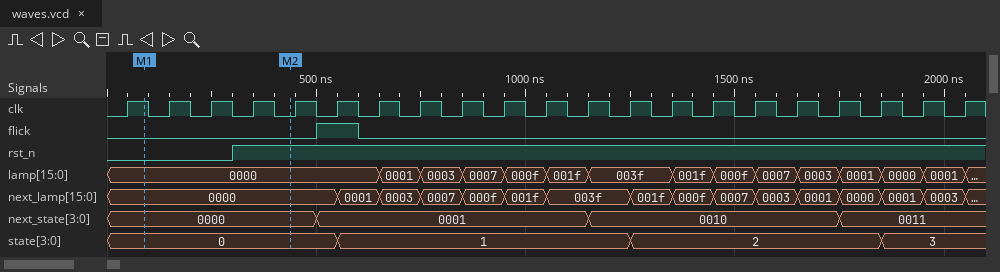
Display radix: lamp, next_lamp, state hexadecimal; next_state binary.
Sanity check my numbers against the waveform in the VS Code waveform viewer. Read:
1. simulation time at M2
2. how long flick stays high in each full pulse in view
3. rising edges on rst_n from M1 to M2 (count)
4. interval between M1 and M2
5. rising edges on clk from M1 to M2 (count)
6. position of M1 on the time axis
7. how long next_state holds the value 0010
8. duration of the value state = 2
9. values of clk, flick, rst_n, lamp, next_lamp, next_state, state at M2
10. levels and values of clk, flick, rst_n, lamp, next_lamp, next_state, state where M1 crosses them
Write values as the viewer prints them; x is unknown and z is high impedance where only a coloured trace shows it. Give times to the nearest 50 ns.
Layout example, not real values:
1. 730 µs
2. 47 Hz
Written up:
1. 450 ns
2. 100 ns
3. 1
4. 350 ns
5. 3
6. 100 ns
7. 600 ns
8. 600 ns
9. clk=0, flick=0, rst_n=1, lamp=0000, next_lamp=0000, next_state=0000, state=0
10. clk=1, flick=0, rst_n=0, lamp=0000, next_lamp=0000, next_state=0000, state=0
